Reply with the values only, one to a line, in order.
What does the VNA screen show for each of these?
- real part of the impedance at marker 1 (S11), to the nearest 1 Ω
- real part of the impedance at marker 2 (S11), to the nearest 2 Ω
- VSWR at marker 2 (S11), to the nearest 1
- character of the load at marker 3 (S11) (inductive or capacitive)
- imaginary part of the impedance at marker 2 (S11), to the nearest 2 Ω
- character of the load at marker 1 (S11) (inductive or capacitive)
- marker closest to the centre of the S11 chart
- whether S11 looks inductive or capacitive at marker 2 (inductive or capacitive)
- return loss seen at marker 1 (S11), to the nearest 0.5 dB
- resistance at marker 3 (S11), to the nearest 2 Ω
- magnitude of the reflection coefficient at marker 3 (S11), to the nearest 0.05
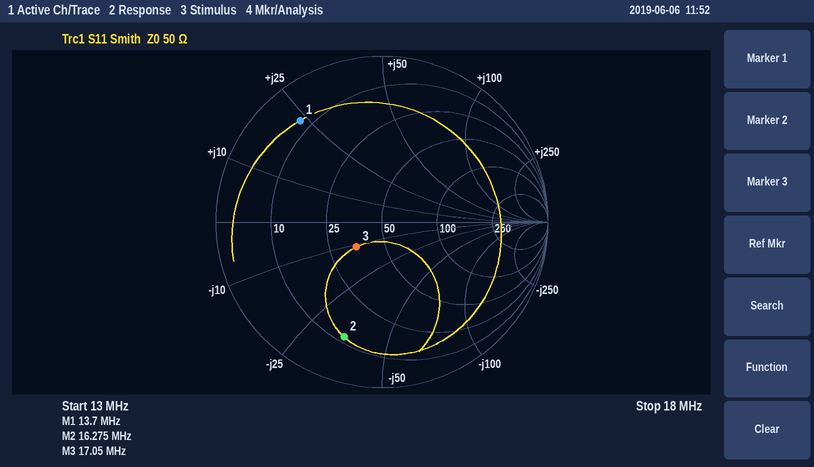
7 Ω
12 Ω
6
capacitive
-34 Ω
inductive
marker 3
capacitive
2.0 dB
36 Ω
0.20
